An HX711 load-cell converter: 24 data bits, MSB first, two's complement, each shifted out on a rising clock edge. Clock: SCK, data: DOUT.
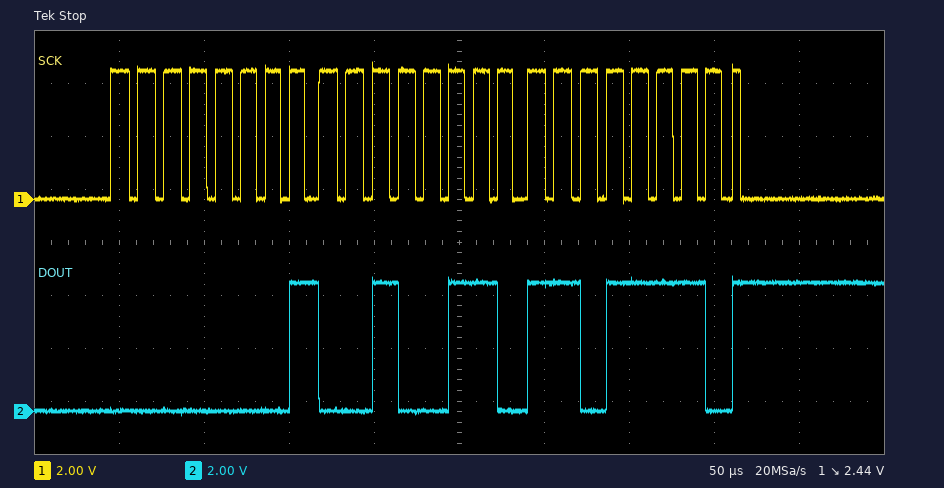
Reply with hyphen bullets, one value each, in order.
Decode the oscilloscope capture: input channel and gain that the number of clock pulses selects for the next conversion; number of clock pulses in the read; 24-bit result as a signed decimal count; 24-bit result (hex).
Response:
- channel A, gain 128
- 25
- 75486
- 0x0126DE
